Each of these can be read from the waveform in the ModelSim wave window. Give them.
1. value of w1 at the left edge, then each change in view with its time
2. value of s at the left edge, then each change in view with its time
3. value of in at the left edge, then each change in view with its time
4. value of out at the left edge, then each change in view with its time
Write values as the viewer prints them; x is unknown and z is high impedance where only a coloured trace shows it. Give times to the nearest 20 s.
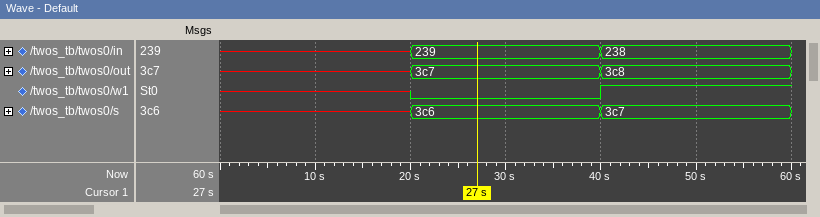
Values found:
x, 0 at 20 s, 1 at 40 s
x, 3c6 at 20 s, 3c7 at 40 s
x, 239 at 20 s, 238 at 40 s
x, 3c7 at 20 s, 3c8 at 40 s
